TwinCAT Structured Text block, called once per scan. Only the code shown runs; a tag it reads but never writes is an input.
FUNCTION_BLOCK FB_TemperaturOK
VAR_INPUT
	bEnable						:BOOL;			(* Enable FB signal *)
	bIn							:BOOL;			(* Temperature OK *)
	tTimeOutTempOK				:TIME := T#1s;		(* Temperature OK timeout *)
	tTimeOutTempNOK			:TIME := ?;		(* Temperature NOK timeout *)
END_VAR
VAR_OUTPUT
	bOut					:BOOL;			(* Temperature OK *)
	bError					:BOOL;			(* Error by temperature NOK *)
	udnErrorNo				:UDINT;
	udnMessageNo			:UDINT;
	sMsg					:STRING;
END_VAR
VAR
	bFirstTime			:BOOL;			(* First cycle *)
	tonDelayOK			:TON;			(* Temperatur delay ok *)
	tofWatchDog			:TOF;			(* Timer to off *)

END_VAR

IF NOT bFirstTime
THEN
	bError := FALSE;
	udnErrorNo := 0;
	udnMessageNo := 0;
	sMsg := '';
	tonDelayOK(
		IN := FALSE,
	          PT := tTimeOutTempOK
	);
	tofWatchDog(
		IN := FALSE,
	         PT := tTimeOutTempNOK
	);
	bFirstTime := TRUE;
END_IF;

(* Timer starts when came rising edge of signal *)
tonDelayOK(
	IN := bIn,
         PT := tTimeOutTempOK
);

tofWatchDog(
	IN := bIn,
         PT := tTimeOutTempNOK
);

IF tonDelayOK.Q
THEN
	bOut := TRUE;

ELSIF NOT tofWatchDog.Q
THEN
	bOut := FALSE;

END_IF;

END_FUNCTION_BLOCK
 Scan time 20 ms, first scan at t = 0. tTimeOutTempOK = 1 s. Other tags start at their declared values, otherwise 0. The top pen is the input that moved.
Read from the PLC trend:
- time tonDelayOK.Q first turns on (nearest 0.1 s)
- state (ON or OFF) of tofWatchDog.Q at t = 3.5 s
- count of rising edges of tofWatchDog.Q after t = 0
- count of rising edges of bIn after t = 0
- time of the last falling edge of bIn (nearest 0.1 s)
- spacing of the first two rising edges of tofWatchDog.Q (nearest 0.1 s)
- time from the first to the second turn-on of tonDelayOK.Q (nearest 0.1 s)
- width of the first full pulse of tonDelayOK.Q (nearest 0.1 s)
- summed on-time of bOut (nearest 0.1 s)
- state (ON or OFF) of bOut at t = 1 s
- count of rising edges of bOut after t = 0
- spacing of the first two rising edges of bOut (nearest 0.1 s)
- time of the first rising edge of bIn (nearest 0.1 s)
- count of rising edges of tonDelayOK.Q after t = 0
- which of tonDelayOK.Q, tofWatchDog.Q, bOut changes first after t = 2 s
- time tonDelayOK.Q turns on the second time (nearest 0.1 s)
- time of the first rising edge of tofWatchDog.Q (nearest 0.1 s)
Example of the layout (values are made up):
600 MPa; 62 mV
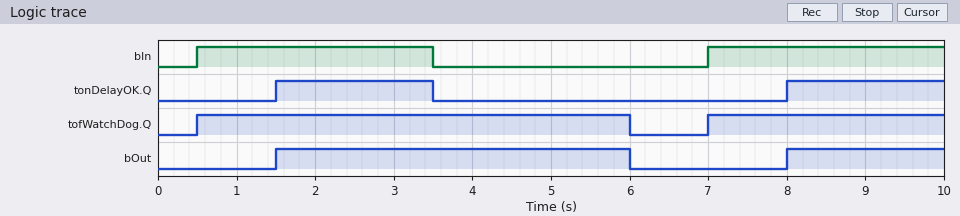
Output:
1.5 s; ON; 2; 2; 3.5 s; 6.5 s; 6.5 s; 2.0 s; 6.5 s; OFF; 2; 6.5 s; 0.5 s; 2; tonDelayOK.Q; 8.0 s; 0.5 s
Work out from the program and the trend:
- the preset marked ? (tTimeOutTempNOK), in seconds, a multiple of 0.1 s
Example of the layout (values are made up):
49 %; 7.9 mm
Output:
2.5 s
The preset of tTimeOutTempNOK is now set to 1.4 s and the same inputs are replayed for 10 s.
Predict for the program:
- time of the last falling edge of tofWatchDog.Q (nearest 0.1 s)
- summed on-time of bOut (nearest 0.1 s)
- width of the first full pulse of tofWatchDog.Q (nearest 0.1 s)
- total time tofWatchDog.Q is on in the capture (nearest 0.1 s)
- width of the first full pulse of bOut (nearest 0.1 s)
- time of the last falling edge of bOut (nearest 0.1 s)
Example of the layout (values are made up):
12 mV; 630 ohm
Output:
4.9 s; 5.4 s; 4.4 s; 7.4 s; 3.4 s; 4.9 s
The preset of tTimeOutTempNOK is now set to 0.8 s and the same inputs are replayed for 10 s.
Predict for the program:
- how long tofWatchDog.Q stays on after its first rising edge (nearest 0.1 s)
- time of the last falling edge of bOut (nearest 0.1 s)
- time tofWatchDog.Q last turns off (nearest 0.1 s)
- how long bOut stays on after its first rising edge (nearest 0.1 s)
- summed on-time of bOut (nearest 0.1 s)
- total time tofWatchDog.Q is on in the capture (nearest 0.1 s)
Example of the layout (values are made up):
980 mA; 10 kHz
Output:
3.8 s; 4.3 s; 4.3 s; 2.8 s; 4.8 s; 6.8 s
